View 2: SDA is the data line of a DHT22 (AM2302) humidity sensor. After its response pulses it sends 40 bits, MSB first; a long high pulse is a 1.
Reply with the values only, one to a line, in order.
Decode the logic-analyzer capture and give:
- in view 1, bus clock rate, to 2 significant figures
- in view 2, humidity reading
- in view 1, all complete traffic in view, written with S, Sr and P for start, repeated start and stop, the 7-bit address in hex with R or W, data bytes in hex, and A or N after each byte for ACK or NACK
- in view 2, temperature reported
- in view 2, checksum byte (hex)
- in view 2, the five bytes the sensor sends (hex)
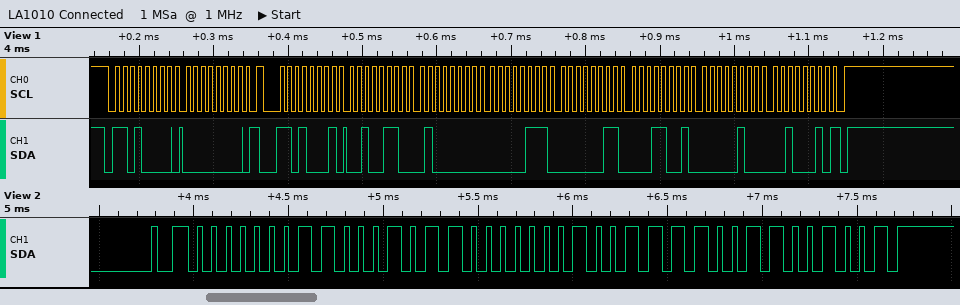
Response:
100 kHz
39.5 %
S 68W A 00 A Sr 68R A 26 A 40 A 07 A 03 A 19 A 04 A 22 N P
31.6 °C
0xC9
01 8B 01 3C C9
